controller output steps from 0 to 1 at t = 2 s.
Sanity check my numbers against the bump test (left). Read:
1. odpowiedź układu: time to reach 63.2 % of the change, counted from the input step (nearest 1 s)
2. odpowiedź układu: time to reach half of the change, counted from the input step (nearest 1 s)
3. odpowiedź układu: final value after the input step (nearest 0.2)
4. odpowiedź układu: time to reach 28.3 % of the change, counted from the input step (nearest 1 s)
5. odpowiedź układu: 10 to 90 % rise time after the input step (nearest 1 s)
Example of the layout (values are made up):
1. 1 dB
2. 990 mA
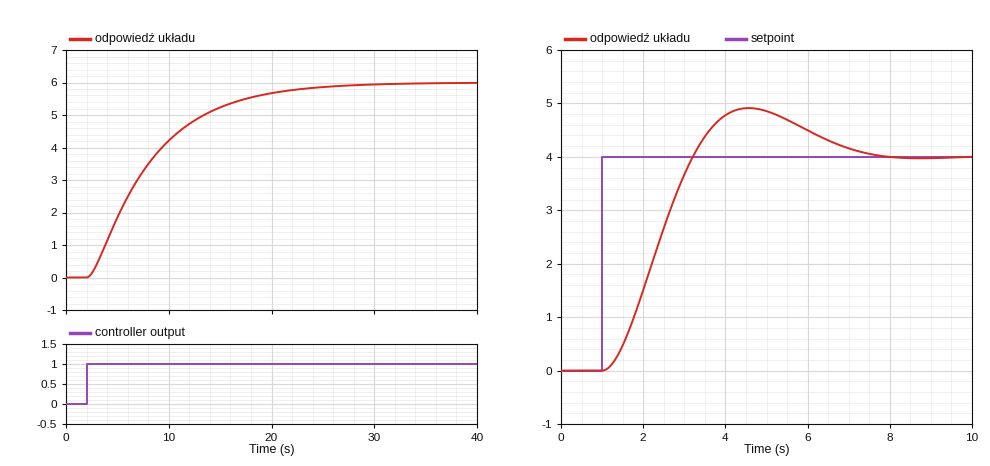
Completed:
1. 7 s
2. 5 s
3. 6.0
4. 3 s
5. 13 s
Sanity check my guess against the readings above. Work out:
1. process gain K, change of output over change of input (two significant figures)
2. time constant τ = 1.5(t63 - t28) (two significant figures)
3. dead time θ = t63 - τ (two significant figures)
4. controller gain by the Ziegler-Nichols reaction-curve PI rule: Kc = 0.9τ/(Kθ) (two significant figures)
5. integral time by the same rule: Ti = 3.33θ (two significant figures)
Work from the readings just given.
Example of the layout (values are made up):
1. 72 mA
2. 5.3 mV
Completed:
1. 6.0
2. 6.0 s
3. 1.0 s
4. 0.90
5. 3.3 s
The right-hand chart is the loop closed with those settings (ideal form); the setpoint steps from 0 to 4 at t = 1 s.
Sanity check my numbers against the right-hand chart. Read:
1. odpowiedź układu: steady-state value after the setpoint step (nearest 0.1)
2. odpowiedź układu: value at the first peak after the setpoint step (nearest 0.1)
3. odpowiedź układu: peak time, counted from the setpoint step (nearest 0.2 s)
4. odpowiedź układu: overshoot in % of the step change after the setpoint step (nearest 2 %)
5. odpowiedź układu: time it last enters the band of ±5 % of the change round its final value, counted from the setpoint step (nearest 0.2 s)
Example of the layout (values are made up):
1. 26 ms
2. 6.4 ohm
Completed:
1. 4.0
2. 4.9
3. 3.6 s
4. 22 %
5. 5.8 s
